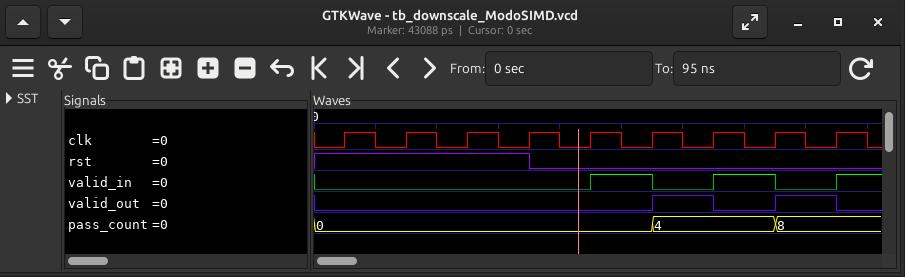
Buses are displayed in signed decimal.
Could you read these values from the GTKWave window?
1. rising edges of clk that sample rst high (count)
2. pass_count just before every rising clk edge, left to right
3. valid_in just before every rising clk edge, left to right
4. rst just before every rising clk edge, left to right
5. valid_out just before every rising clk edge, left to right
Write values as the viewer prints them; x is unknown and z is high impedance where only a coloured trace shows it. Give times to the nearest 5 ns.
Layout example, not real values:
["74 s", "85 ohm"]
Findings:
["4", "0, 0, 0, 0, 0, 0, 4, 4, 8", "0 0 0 0 0 1 0 1 0", "1 1 1 1 0 0 0 0 0", "0 0 0 0 0 0 1 0 1"]
